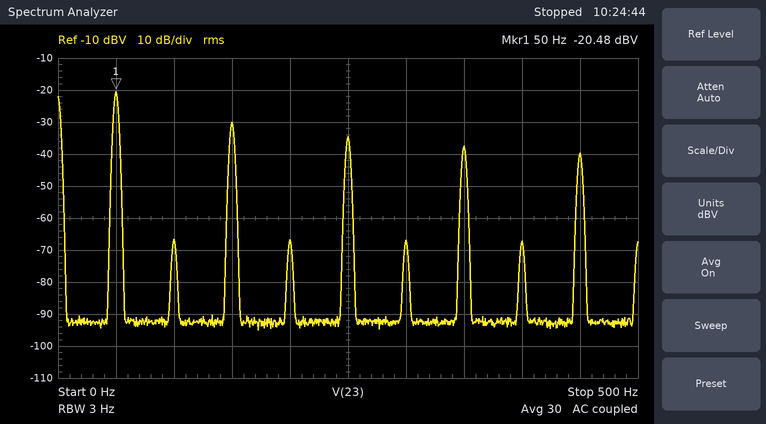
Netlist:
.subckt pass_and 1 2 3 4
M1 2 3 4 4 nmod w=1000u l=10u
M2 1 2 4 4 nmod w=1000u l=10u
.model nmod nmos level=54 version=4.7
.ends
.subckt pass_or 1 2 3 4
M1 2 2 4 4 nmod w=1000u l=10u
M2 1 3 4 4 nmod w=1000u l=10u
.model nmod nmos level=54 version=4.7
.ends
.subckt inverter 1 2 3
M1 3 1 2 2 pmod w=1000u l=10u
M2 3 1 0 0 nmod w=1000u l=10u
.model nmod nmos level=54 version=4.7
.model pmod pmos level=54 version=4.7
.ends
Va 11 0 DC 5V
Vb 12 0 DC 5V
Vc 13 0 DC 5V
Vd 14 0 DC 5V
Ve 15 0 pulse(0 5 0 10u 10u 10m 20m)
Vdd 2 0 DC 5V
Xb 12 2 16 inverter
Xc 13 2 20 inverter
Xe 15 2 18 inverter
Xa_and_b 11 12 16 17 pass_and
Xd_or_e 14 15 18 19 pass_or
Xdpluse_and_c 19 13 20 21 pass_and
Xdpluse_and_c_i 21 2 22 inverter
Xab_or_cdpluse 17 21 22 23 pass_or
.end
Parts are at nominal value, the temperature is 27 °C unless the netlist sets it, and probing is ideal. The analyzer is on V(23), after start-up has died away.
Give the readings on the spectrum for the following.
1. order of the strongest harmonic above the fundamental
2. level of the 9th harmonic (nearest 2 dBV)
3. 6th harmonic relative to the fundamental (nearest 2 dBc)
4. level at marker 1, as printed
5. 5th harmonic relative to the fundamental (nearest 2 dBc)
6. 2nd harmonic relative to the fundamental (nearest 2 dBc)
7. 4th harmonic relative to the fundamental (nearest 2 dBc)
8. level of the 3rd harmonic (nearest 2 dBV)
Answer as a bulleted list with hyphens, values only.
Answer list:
- 3
- -40 dBV
- -46 dBc
- -20.48 dBV
- -14 dBc
- -46 dBc
- -46 dBc
- -30 dBV
